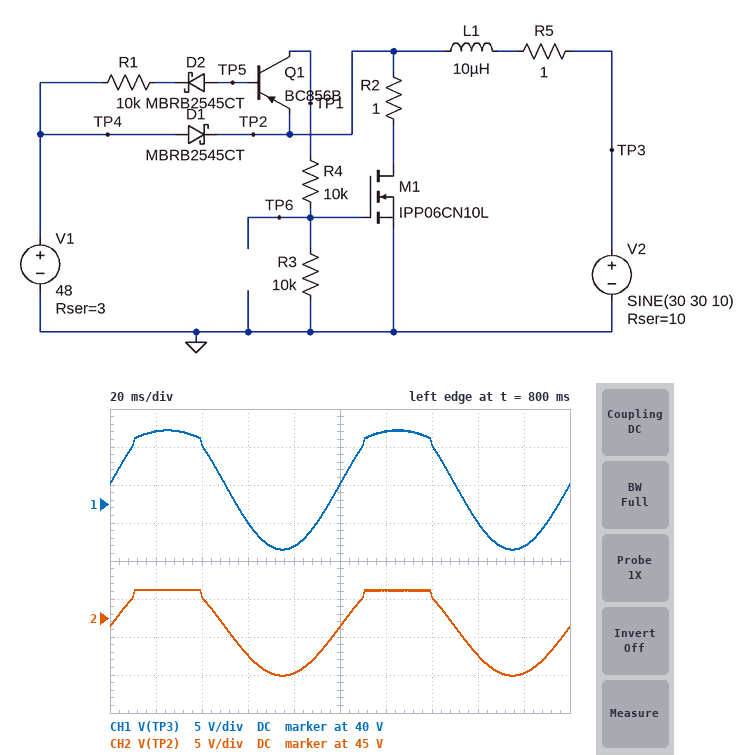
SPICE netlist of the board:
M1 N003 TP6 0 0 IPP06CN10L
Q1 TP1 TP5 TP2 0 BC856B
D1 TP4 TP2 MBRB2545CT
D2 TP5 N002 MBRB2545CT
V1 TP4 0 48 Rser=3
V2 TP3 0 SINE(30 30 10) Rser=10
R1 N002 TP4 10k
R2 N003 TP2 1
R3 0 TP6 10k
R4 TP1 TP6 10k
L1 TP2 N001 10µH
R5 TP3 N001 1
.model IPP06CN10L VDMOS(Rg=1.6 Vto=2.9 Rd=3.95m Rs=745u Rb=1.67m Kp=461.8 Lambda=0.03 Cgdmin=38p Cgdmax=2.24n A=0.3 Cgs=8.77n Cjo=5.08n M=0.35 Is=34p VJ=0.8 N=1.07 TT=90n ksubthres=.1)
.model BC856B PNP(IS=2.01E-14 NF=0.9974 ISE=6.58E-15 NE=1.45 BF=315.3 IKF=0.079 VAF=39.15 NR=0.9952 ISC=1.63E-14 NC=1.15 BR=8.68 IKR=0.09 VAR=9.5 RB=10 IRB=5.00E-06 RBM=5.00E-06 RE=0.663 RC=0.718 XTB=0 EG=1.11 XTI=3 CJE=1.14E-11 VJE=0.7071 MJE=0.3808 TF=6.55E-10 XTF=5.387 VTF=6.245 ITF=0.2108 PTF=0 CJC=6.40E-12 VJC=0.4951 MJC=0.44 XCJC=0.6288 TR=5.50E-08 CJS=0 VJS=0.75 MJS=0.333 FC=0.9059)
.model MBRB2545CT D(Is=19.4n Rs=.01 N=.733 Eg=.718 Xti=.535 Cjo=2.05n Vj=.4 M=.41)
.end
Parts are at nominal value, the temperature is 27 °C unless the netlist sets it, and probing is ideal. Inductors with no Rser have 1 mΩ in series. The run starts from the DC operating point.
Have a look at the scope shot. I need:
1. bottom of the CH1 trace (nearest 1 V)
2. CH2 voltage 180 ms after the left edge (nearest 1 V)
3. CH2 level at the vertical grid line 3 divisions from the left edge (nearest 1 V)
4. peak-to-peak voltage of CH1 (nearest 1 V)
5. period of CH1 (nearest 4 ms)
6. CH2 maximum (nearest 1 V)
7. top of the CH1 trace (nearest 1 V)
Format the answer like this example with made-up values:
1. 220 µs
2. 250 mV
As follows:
1. 34 V
2. 38 V
3. 40 V
4. 16 V
5. 100 ms
6. 49 V
7. 50 V
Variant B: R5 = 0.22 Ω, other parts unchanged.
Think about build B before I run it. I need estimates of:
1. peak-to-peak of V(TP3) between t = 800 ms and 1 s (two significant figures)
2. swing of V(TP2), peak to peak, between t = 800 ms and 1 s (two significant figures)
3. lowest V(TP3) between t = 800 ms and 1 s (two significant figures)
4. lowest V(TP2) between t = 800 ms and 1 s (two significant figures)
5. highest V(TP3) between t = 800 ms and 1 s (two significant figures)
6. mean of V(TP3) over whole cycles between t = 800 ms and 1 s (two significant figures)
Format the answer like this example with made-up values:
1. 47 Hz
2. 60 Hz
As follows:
1. 13 V
2. 12 V
3. 36 V
4. 37 V
5. 49 V
6. 43 V
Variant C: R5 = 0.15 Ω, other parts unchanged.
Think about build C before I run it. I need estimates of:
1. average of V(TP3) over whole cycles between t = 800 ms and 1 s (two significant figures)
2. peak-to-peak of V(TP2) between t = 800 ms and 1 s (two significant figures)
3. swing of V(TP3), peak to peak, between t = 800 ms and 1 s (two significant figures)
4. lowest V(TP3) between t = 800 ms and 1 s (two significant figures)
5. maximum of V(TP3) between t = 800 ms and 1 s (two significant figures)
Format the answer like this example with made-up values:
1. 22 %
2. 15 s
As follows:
1. 43 V
2. 12 V
3. 13 V
4. 36 V
5. 49 V
